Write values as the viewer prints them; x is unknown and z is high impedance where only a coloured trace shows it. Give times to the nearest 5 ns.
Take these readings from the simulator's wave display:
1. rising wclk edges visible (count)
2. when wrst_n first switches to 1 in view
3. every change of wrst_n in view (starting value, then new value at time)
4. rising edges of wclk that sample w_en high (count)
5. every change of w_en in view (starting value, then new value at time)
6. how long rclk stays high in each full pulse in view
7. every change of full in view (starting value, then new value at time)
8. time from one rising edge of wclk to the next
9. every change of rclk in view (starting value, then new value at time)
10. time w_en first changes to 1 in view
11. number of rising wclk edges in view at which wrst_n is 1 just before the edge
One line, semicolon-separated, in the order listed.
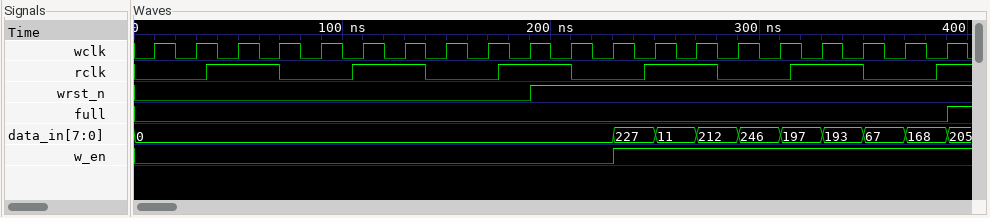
20; 190 ns; 0, 1 at 190 ns; 8; 0, 1 at 230 ns; 35 ns, 35 ns, 35 ns, 35 ns, 35 ns; 0, 1 at 390 ns; 20 ns; 0, 1 at 35 ns, 0 at 70 ns, 1 at 105 ns, 0 at 140 ns, 1 at 175 ns, 0 at 210 ns, 1 at 245 ns, 0 at 280 ns, 1 at 315 ns, 0 at 350 ns, 1 at 385 ns; 230 ns; 10
